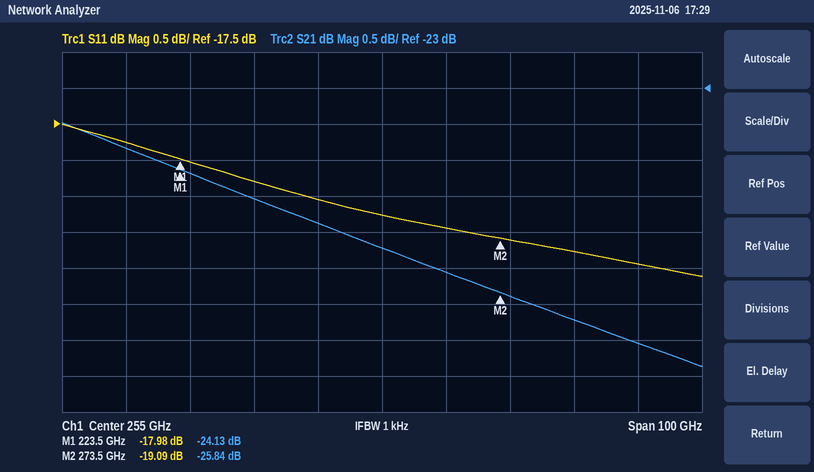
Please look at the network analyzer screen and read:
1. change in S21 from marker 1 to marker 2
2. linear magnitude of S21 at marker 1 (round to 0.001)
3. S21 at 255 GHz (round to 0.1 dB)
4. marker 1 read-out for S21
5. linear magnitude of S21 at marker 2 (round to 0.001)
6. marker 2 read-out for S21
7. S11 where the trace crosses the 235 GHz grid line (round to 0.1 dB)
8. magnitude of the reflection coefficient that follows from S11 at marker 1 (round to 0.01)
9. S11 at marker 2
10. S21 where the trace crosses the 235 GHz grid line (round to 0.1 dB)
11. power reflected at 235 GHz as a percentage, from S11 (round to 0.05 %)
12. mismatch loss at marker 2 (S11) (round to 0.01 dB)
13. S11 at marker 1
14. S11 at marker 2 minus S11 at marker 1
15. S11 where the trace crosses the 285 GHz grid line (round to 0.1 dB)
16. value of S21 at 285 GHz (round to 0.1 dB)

-1.71 dB
0.062
-25.2 dB
-24.13 dB
0.051
-25.84 dB
-18.3 dB
0.13
-19.09 dB
-24.5 dB
1.50 %
0.05 dB
-17.98 dB
-1.11 dB
-19.3 dB
-26.2 dB
